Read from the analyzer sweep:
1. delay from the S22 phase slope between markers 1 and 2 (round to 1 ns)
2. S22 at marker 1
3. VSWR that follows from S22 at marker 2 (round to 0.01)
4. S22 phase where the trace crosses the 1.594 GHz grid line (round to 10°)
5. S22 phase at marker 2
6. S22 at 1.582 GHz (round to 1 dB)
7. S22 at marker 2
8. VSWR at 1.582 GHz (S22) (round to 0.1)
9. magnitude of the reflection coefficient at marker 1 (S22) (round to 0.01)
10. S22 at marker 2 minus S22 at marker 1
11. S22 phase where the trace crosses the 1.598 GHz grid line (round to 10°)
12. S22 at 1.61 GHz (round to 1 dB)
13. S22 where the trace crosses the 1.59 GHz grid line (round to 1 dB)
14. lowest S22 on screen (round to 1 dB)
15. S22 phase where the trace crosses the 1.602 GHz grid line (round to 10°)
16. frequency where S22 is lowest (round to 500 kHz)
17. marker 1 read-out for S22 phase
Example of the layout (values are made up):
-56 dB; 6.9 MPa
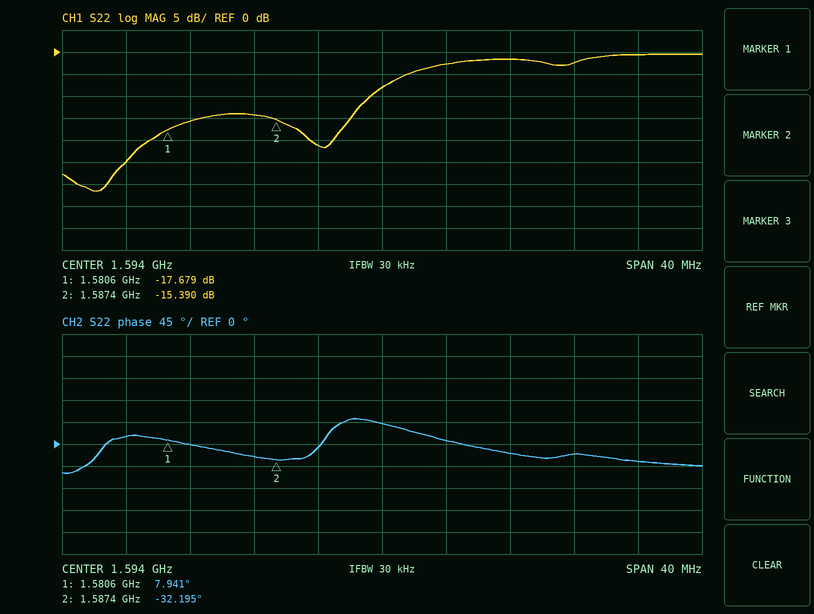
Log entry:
16 ns; -17.679 dB; 1.41; 40°; -32.195°; -16 dB; -15.390 dB; 1.4; 0.13; 2.289 dB; 10°; -1 dB; -21 dB; -32 dB; -20°; 1.5760 GHz; 7.941°
